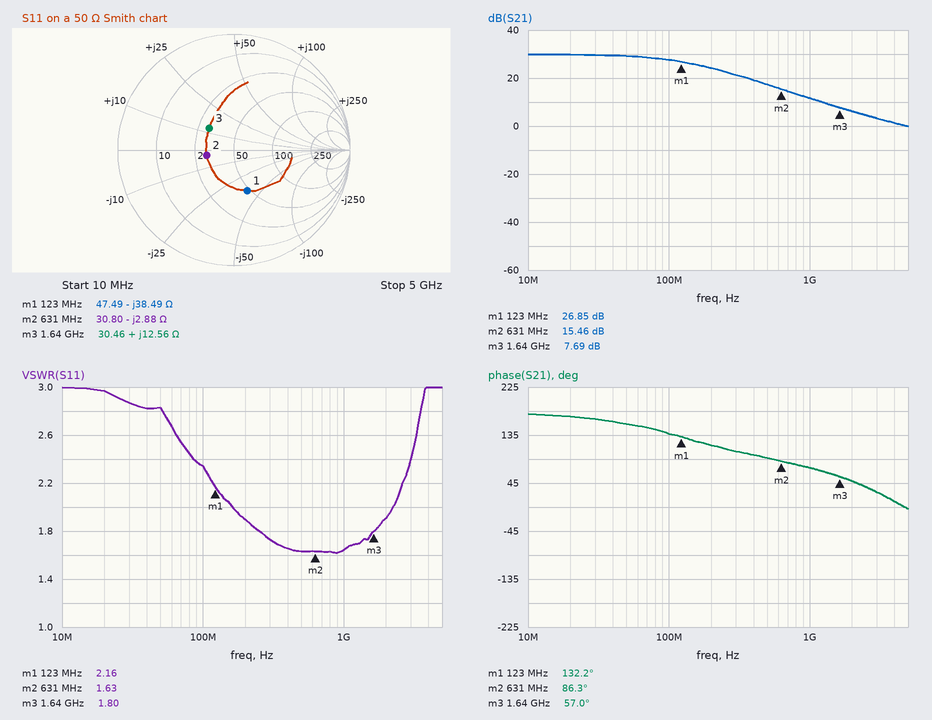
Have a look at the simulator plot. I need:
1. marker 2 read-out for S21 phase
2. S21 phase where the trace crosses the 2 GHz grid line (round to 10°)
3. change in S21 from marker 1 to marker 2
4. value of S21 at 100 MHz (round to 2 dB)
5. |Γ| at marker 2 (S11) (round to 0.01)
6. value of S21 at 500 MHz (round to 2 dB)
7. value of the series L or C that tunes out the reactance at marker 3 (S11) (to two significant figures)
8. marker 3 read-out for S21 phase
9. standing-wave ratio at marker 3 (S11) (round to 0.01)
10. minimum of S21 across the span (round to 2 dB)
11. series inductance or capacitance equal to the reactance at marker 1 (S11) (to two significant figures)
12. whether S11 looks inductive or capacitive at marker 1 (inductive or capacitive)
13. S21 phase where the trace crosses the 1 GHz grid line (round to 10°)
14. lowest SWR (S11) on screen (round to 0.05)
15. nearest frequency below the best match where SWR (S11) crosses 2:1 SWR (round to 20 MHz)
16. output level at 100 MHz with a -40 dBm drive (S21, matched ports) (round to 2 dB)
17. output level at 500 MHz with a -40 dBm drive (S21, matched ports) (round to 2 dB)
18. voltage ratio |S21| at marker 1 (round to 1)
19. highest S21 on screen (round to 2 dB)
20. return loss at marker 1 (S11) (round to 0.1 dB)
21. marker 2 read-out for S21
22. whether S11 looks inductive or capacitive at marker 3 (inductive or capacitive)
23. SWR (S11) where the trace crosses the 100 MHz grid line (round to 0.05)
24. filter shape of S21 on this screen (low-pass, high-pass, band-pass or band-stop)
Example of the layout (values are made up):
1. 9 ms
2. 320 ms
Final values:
1. 86.3°
2. 50°
3. -11.39 dB
4. 28 dB
5. 0.24
6. 18 dB
7. 7.7 pF
8. 57.0°
9. 1.80
10. 0 dB
11. 34 pF
12. capacitive
13. 70°
14. 1.60
15. 160 MHz
16. -12 dBm
17. -22 dBm
18. 22
19. 30 dB
20. 8.7 dB
21. 15.46 dB
22. inductive
23. 2.35
24. low-pass
